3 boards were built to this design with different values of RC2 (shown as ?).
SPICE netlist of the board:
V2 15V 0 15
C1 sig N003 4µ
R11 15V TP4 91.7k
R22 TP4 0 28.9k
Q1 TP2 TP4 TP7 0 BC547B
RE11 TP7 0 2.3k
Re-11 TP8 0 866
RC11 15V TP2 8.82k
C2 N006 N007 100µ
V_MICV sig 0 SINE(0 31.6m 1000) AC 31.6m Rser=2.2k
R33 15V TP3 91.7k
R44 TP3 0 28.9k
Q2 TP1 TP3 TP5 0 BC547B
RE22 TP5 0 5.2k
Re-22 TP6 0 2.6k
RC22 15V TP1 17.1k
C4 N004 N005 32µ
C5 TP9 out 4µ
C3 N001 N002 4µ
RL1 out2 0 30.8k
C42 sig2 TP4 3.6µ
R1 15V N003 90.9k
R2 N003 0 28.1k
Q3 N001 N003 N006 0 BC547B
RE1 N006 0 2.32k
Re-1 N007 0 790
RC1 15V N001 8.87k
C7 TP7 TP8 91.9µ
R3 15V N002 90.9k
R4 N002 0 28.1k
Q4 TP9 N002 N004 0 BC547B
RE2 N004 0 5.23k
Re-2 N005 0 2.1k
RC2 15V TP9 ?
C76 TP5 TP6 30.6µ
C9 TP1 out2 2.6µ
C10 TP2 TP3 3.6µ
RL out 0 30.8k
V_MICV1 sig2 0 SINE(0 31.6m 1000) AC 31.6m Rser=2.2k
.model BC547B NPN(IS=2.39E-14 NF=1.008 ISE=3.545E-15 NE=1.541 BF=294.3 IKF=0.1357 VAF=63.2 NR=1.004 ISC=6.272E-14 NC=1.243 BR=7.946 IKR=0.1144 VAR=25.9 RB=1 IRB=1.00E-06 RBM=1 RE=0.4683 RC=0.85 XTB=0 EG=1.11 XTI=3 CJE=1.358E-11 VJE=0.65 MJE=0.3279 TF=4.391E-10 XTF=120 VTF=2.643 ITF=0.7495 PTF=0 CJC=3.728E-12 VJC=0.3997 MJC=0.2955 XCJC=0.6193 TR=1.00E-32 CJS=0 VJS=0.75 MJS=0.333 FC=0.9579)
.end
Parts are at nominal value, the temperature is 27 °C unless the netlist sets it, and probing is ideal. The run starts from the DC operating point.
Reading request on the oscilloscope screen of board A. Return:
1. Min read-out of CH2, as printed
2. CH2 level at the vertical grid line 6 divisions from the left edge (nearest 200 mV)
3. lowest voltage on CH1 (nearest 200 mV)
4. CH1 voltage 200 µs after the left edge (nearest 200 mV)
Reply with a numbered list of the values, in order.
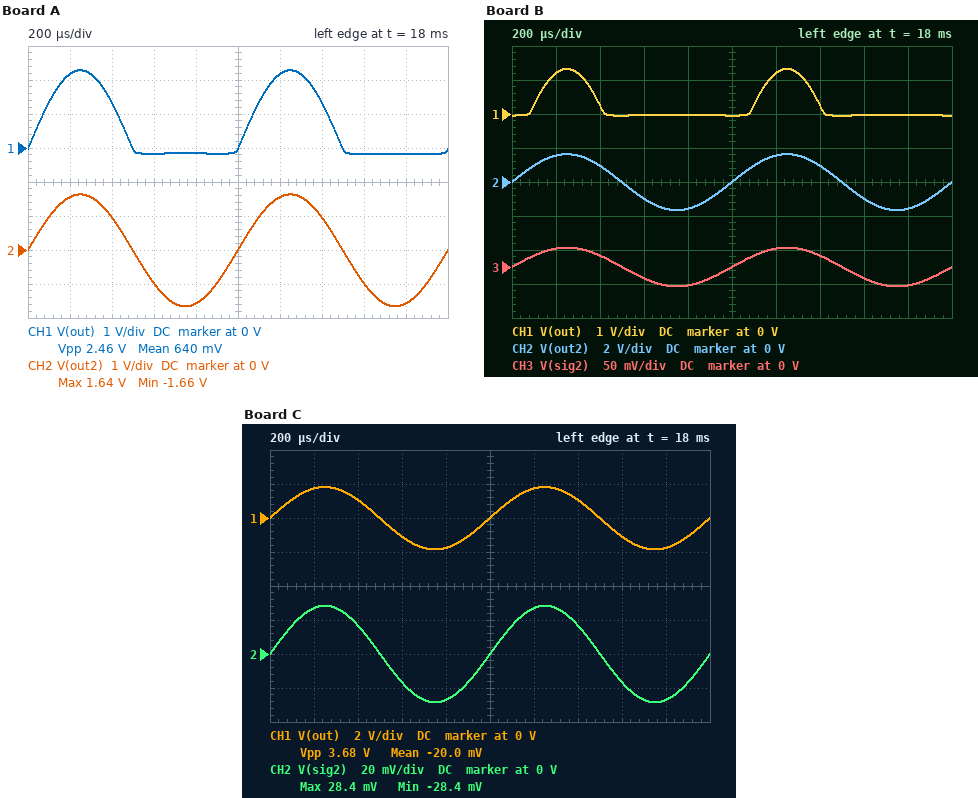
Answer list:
1. -1.66 V
2. 1.6 V
3. -200 mV
4. 2.2 V
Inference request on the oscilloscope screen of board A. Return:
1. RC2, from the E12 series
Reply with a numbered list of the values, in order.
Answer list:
1. 22 kΩ
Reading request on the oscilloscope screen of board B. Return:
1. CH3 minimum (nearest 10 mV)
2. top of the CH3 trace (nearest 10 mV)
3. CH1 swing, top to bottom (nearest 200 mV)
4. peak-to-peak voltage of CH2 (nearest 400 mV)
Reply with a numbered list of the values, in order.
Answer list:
1. -30 mV
2. 30 mV
3. 1.4 V
4. 3.2 V
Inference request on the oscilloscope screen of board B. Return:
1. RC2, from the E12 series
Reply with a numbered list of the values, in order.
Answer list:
1. 27 kΩ
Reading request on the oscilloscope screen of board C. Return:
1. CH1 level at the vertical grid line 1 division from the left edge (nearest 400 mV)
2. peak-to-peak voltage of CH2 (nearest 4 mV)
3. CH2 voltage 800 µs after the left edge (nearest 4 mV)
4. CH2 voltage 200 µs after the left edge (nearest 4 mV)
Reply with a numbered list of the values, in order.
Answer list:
1. 1.6 V
2. 56 mV
3. -28 mV
4. 28 mV
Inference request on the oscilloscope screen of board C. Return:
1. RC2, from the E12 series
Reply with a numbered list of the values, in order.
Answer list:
1. 15 kΩ
